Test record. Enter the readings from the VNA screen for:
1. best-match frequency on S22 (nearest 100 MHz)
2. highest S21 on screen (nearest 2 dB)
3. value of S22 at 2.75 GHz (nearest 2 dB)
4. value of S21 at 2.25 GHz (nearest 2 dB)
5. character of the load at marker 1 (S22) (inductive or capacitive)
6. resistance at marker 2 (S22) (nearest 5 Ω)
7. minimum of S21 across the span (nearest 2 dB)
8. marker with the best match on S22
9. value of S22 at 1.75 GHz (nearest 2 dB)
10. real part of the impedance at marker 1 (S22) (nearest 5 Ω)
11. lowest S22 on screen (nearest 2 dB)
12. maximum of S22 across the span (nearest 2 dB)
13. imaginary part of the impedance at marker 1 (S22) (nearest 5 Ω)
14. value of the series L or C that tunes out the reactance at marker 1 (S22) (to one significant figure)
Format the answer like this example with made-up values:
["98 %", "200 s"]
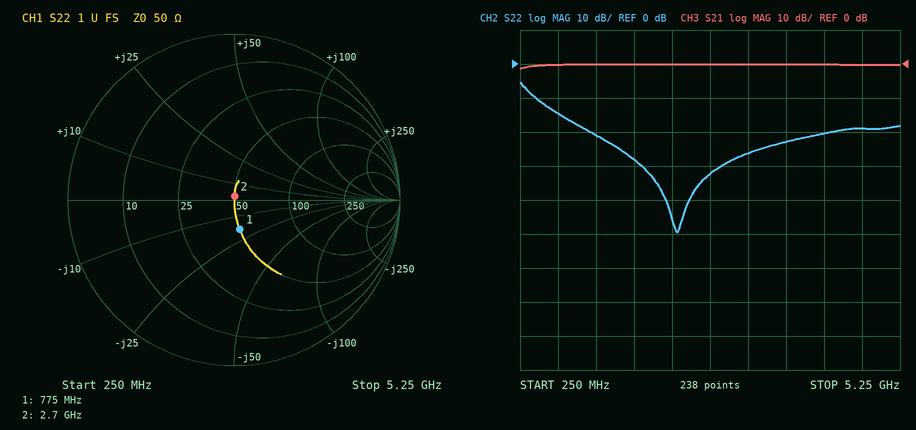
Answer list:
["2.3 GHz", "0 dB", "-32 dB", "0 dB", "capacitive", "50 Ω", "-2 dB", "marker 2", "-28 dB", "50 Ω", "-50 dB", "-6 dB", "-20 Ω", "4 nH"]
